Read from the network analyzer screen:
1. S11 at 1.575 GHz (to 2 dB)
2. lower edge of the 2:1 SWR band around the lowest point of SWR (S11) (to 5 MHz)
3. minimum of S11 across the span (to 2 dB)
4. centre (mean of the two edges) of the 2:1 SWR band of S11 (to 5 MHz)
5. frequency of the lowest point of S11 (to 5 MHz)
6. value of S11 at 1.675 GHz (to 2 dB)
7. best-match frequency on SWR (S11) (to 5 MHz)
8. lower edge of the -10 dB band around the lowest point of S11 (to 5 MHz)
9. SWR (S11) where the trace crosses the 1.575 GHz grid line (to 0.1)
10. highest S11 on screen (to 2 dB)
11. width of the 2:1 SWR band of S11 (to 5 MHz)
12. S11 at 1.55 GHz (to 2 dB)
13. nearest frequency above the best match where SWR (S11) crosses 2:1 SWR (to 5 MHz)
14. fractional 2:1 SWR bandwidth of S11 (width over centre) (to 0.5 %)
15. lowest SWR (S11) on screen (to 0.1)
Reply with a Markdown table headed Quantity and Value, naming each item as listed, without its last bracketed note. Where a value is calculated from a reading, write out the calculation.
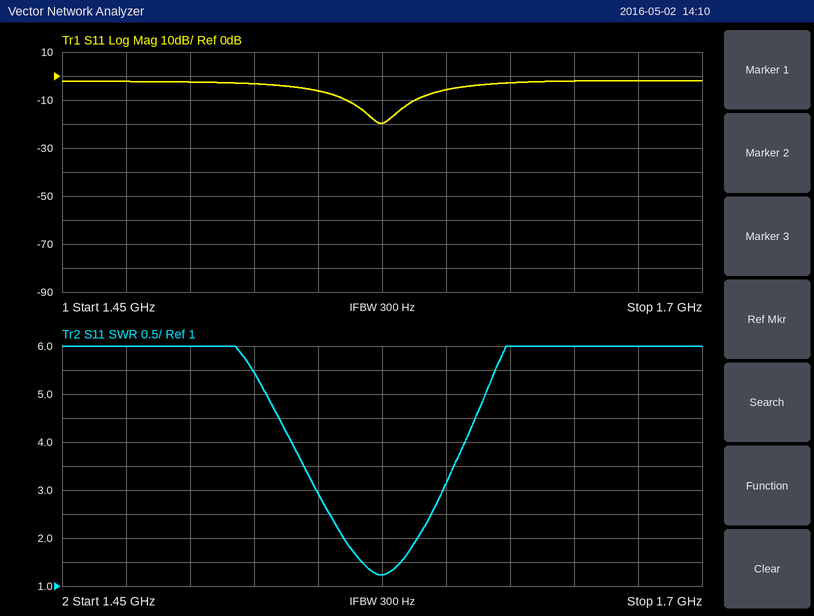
| Quantity | Value |
|---|---|
| S11 at 1.575 GHz | -20 dB |
| lower edge of the 2:1 SWR band around the lowest point of SWR (S11) | 1.560 GHz |
| minimum of S11 across the span | -20 dB |
| centre (mean of the two edges) of the 2:1 SWR band of S11 | 1.575 GHz |
| frequency of the lowest point of S11 | 1.575 GHz |
| value of S11 at 1.675 GHz | -2 dB |
| best-match frequency on SWR (S11) | 1.575 GHz |
| lower edge of the -10 dB band around the lowest point of S11 | 1.560 GHz |
| SWR (S11) where the trace crosses the 1.575 GHz grid line | 1.2 |
| highest S11 on screen | -2 dB |
| width of the 2:1 SWR band of S11 | 1.590 GHz − 1.560 GHz = 30 MHz |
| S11 at 1.55 GHz | -6 dB |
| nearest frequency above the best match where SWR (S11) crosses 2:1 SWR | 1.590 GHz |
| fractional 2:1 SWR bandwidth of S11 (width over centre) | 30 MHz / 1.575 GHz ≈ 1.90 %, so 2.0 % to the nearest 0.5 % |
| lowest SWR (S11) on screen | 1.2 |
